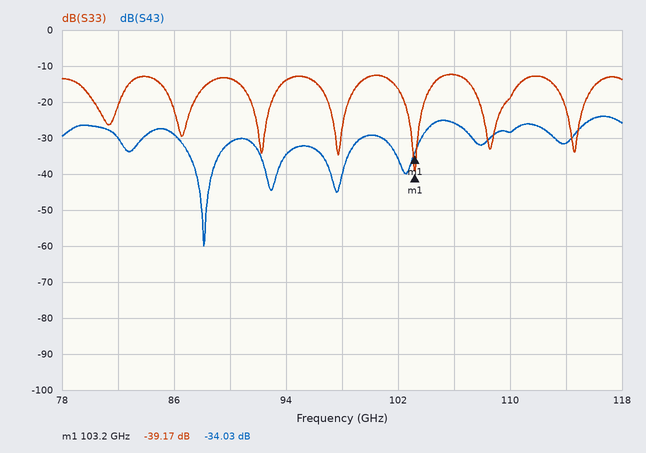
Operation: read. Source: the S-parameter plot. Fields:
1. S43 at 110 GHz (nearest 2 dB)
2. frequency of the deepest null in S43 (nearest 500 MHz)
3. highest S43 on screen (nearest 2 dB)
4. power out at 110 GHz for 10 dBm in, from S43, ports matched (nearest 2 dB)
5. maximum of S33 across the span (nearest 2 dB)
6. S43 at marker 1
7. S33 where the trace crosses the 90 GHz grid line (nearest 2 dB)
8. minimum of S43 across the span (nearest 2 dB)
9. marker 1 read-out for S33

-28 dB
88.0 GHz
-24 dB
-18 dBm
-12 dB
-34.03 dB
-14 dB
-60 dB
-39.17 dB
